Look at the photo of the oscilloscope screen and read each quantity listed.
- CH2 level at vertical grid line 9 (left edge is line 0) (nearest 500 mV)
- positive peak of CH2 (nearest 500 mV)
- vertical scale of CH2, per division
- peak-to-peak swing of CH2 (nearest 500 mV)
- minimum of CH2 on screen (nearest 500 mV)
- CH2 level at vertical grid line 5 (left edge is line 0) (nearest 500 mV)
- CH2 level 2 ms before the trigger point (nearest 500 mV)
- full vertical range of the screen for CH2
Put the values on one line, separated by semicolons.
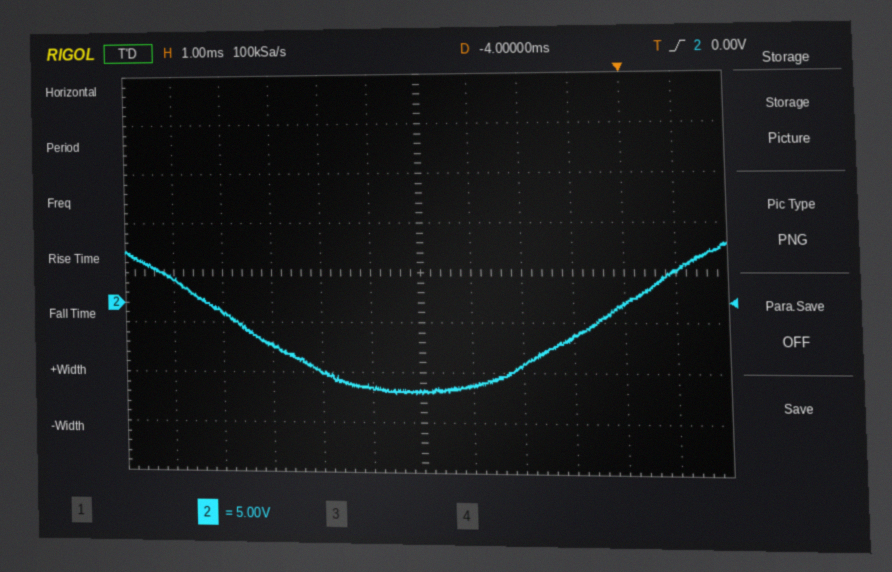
-3.5 V; 6.0 V; 5 V; 15.0 V; -9.0 V; -8.5 V; -6.0 V; 40 V
